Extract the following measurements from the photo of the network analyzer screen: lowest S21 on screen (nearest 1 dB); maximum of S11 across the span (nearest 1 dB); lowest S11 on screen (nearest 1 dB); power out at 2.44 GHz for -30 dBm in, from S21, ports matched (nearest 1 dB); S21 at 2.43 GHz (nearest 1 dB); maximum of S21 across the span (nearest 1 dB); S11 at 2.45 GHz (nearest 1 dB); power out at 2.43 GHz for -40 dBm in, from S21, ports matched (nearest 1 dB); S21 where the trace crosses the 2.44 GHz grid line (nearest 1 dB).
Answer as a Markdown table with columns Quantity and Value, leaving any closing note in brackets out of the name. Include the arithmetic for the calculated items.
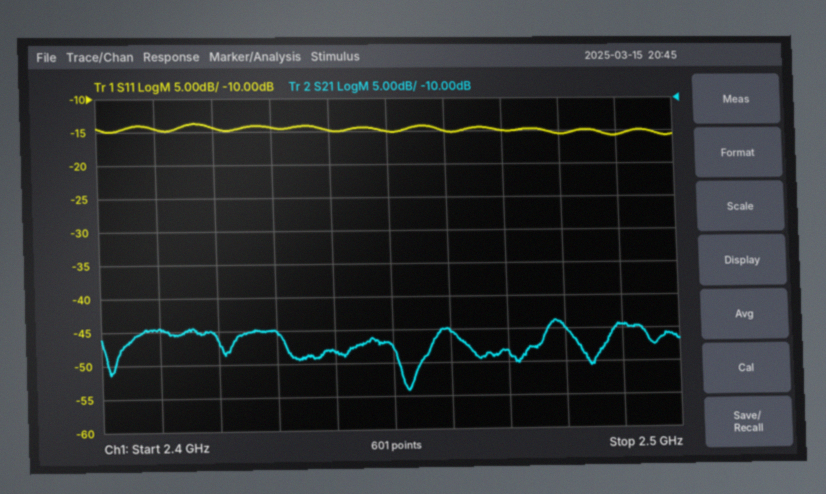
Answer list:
| Quantity | Value |
|---|---|
| lowest S21 on screen | -54 dB |
| maximum of S11 across the span | -14 dB |
| lowest S11 on screen | -16 dB |
| power out at 2.44 GHz for -30 dBm in, from S21, ports matched | -30 dBm + (-48 dB) = -78 dBm |
| S21 at 2.43 GHz | -45 dB |
| maximum of S21 across the span | -44 dB |
| S11 at 2.45 GHz | -15 dB |
| power out at 2.43 GHz for -40 dBm in, from S21, ports matched | -40 dBm + (-45 dB) = -85 dBm |
| S21 where the trace crosses the 2.44 GHz grid line | -48 dB |
